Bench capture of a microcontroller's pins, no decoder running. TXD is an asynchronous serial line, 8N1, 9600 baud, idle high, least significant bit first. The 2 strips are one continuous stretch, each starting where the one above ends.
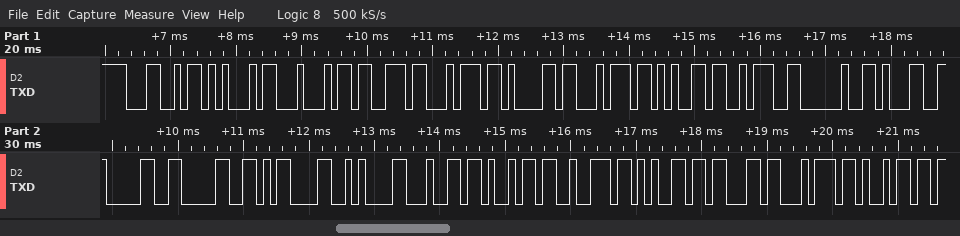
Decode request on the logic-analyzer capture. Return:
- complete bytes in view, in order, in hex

0x4C 0x45 0x44 0x73 0x74 0x61 0x74 0x65 0x3A 0x20 0x31 0x30 0x30 0x0D 0x0A 0x64 0x69 0x72 0x65 0x63 0x74 0x69
